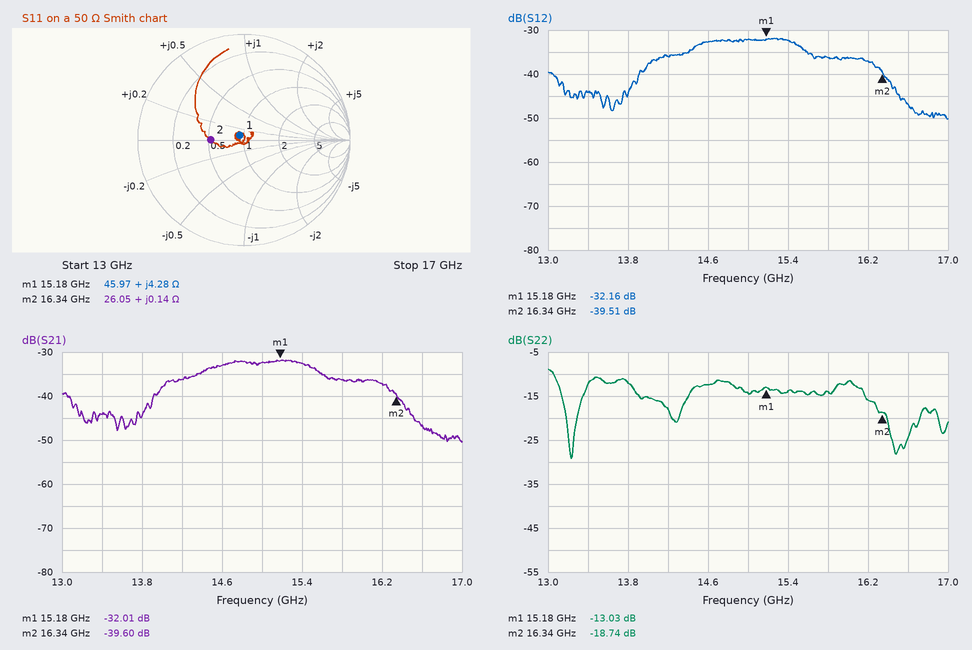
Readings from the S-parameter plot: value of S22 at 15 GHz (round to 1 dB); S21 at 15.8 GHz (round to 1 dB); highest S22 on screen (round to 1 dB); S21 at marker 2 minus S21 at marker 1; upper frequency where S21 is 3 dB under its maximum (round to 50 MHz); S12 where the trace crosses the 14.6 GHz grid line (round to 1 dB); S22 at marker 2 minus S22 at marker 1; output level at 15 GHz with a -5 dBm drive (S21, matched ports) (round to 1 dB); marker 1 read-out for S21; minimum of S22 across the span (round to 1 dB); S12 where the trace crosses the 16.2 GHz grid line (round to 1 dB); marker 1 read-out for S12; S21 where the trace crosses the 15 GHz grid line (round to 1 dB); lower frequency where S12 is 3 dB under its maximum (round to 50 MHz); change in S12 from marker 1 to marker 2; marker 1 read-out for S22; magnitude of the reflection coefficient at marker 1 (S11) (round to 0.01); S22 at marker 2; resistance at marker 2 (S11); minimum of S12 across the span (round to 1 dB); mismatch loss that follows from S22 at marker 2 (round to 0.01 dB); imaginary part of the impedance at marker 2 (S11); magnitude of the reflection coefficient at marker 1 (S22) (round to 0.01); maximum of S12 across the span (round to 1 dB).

-14 dB
-36 dB
-9 dB
-7.59 dB
15.60 GHz
-33 dB
-5.71 dB
-37 dBm
-32.01 dB
-29 dB
-37 dB
-32.16 dB
-32 dB
14.40 GHz
-7.35 dB
-13.03 dB
0.06
-18.74 dB
26.05 Ω
-50 dB
0.06 dB
+0.14 Ω
0.22
-32 dB
